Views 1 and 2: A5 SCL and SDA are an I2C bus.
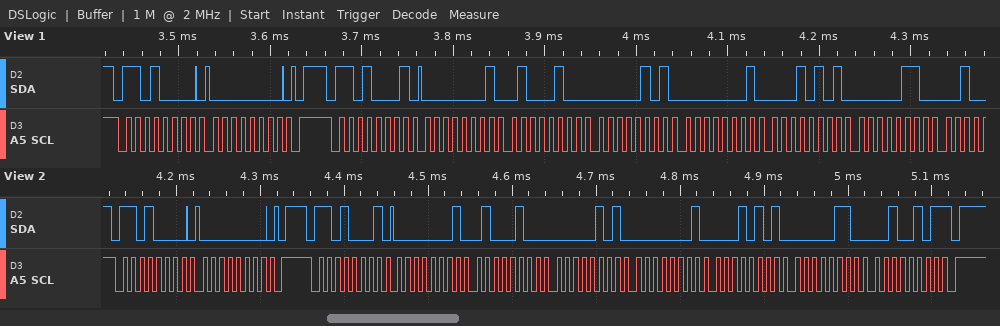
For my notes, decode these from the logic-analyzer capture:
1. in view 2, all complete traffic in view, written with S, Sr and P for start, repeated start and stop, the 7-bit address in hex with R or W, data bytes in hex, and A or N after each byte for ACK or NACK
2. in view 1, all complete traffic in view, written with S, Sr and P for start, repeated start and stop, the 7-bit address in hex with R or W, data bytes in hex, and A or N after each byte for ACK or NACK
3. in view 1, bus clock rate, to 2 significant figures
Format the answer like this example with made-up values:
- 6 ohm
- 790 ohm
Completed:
- S 68W A 00 A P S 68R A 01 A 44 A 05 A 01 A 15 A 06 A 25 N P
- S 68W A 00 A P S 68R A 01 A 44 A 05 A 01 A 15 A 06 A
- 100 kHz
